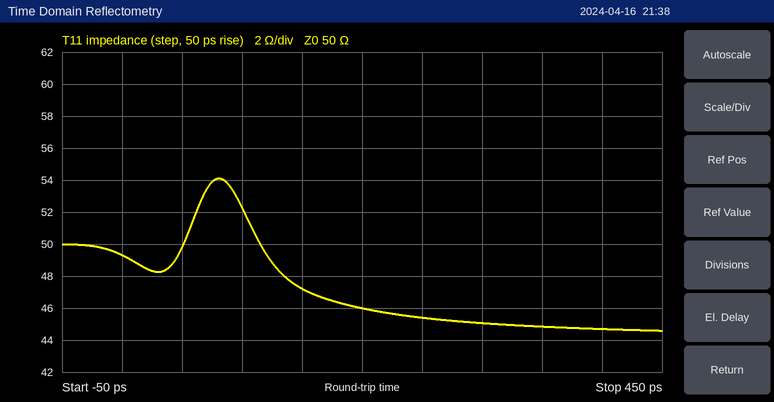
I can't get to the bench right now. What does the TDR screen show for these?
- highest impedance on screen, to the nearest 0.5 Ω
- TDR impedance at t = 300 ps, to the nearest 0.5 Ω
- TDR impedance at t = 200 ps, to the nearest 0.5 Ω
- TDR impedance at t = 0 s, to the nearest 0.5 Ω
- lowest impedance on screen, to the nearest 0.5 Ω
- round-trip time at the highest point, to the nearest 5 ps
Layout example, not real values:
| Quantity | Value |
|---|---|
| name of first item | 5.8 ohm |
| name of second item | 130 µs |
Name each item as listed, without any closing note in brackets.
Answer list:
| Quantity | Value |
|---|---|
| highest impedance on screen, to the nearest 0.5 Ω | 54.0 Ω |
| TDR impedance at t = 300 ps, to the nearest 0.5 Ω | 45.0 Ω |
| TDR impedance at t = 200 ps, to the nearest 0.5 Ω | 46.0 Ω |
| TDR impedance at t = 0 s, to the nearest 0.5 Ω | 49.5 Ω |
| lowest impedance on screen, to the nearest 0.5 Ω | 44.5 Ω |
| round-trip time at the highest point, to the nearest 5 ps | 80 ps |
